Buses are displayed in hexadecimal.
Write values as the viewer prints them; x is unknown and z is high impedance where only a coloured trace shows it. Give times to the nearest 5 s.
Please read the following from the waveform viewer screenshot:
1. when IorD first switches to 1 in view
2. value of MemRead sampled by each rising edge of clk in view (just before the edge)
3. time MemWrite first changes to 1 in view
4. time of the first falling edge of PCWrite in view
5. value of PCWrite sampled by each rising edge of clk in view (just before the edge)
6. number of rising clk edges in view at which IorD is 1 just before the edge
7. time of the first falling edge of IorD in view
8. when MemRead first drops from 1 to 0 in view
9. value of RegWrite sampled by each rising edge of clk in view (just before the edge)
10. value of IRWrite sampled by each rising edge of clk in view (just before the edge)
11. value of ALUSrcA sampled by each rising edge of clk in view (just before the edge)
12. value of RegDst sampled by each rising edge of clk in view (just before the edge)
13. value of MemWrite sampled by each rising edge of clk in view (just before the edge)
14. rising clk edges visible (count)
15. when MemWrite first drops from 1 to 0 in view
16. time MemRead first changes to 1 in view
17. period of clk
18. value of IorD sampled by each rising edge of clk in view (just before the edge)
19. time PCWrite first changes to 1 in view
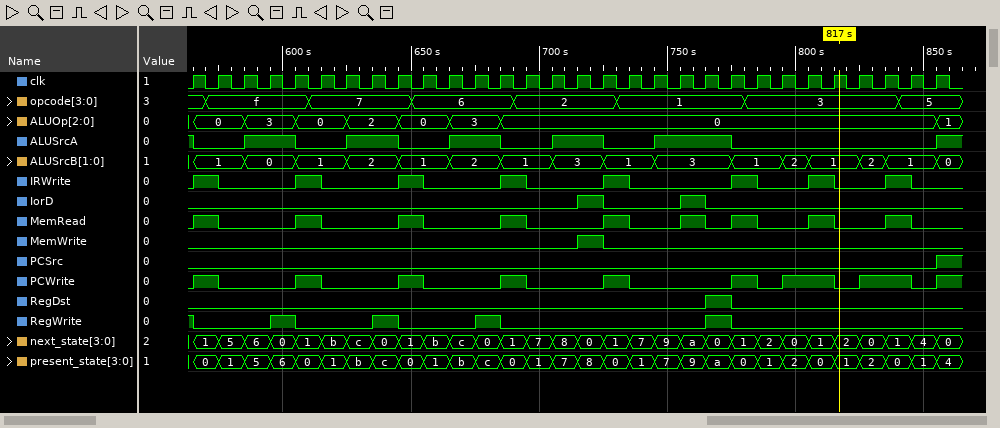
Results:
715 s
0 1 0 0 0 1 0 0 0 1 0 0 0 1 0 0 0 1 0 0 1 0 1 0 0 1 0 0 1 0
715 s
575 s
0 1 0 0 0 1 0 0 0 1 0 0 0 1 0 0 0 1 0 0 0 0 1 0 1 1 0 1 1 0
2
725 s
575 s
1 0 0 0 1 0 0 0 1 0 0 0 1 0 0 0 0 0 0 0 0 1 0 0 0 0 0 0 0 0
0 1 0 0 0 1 0 0 0 1 0 0 0 1 0 0 0 1 0 0 0 0 1 0 0 1 0 0 1 0
1 0 0 1 1 0 0 1 1 0 0 1 1 0 0 1 1 0 0 1 1 1 0 0 0 0 0 0 0 0
0 0 0 0 0 0 0 0 0 0 0 0 0 0 0 0 0 0 0 0 0 1 0 0 0 0 0 0 0 0
0 0 0 0 0 0 0 0 0 0 0 0 0 0 0 0 1 0 0 0 0 0 0 0 0 0 0 0 0 0
30
725 s
565 s
10 s
0 0 0 0 0 0 0 0 0 0 0 0 0 0 0 0 1 0 0 0 1 0 0 0 0 0 0 0 0 0
565 s
